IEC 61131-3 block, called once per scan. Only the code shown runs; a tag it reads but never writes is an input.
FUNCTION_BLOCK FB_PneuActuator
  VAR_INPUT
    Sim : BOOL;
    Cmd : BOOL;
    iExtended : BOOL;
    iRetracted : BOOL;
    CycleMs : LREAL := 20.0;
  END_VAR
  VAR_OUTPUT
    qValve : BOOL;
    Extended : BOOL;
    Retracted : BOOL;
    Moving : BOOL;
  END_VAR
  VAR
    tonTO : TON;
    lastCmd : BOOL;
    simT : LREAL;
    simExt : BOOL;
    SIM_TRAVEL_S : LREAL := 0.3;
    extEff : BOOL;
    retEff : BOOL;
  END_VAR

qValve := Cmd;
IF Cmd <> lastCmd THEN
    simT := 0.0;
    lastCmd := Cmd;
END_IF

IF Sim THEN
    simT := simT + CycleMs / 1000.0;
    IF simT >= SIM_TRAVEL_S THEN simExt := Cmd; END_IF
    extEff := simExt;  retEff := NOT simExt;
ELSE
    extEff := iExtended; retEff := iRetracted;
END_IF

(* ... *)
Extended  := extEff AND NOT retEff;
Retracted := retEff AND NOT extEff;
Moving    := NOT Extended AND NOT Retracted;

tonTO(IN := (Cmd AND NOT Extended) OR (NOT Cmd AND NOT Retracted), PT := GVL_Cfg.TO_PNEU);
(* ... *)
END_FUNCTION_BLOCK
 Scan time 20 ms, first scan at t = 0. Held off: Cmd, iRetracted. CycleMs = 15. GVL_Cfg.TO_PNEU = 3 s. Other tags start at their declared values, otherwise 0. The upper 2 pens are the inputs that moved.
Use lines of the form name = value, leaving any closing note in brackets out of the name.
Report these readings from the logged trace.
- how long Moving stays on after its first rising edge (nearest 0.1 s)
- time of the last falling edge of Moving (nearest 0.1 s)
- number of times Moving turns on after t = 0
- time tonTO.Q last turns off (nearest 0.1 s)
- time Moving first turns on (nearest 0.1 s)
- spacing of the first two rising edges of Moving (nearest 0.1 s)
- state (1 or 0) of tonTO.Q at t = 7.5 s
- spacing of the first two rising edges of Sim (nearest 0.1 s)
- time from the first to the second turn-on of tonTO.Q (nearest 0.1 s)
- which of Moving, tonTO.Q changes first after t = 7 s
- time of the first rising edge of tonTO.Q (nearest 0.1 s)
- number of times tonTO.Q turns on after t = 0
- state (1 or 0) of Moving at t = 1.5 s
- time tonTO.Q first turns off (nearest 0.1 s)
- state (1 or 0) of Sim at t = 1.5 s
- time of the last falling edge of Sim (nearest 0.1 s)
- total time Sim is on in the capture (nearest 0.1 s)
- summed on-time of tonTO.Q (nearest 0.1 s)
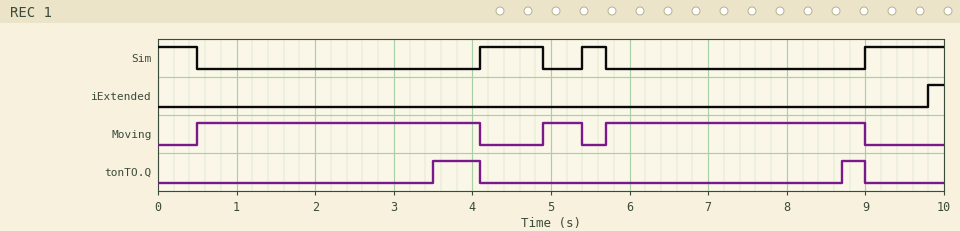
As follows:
how long Moving stays on after its first rising edge = 3.6 s
time of the last falling edge of Moving = 9.0 s
number of times Moving turns on after t = 0 = 3
time tonTO.Q last turns off = 9.0 s
time Moving first turns on = 0.5 s
spacing of the first two rising edges of Moving = 4.4 s
state (1 or 0) of tonTO.Q at t = 7.5 s = 0
spacing of the first two rising edges of Sim = 1.3 s
time from the first to the second turn-on of tonTO.Q = 5.2 s
which of Moving, tonTO.Q changes first after t = 7 s = tonTO.Q
time of the first rising edge of tonTO.Q = 3.5 s
number of times tonTO.Q turns on after t = 0 = 2
state (1 or 0) of Moving at t = 1.5 s = 1
time tonTO.Q first turns off = 4.1 s
state (1 or 0) of Sim at t = 1.5 s = 0
time of the last falling edge of Sim = 5.7 s
total time Sim is on in the capture = 2.6 s
summed on-time of tonTO.Q = 0.9 s
